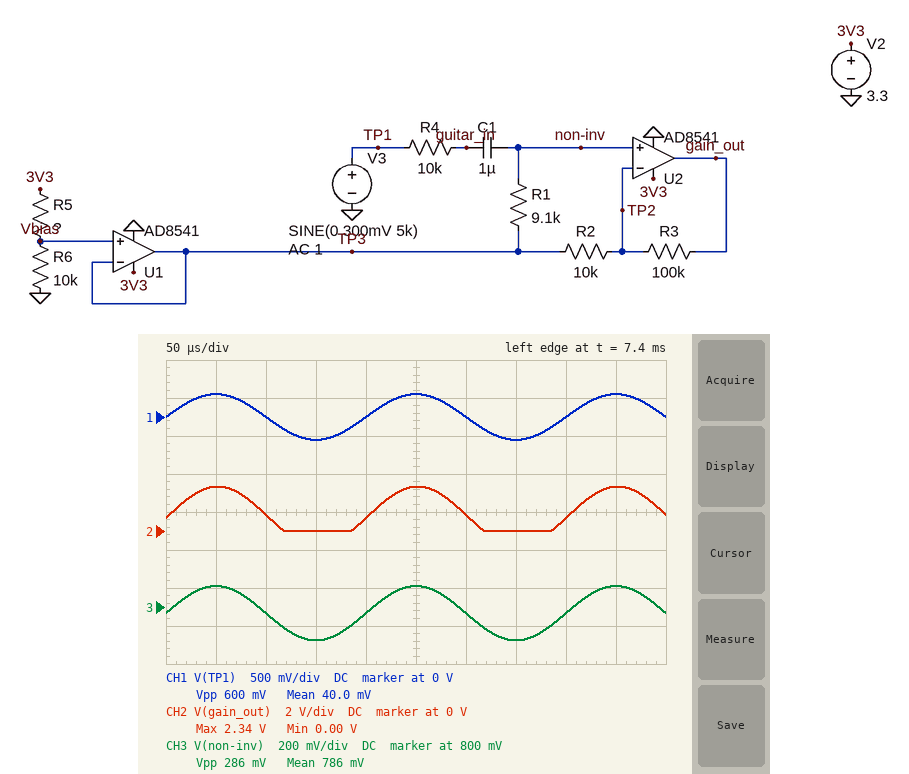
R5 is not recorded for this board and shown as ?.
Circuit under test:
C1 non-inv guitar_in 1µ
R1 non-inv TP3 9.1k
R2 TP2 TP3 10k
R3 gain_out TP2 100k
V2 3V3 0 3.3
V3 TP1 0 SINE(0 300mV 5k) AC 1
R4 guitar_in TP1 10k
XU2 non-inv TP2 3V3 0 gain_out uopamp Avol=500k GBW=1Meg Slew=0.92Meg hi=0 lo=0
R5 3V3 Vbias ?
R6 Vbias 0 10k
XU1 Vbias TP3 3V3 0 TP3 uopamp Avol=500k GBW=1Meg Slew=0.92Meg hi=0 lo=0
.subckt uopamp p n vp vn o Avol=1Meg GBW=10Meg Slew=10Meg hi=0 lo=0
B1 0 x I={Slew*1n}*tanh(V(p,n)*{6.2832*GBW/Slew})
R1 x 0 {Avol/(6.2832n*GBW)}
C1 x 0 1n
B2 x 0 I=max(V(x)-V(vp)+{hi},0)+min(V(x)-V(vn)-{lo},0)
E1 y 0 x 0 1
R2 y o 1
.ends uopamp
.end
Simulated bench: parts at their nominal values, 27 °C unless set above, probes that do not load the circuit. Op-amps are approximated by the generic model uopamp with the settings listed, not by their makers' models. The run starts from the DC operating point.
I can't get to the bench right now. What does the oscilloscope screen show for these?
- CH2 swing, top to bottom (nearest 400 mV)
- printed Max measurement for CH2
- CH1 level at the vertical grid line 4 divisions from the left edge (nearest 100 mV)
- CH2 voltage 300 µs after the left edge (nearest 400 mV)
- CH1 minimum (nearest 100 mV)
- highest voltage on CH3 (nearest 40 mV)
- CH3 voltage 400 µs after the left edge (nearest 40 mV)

2.4 V
2.34 V
0 V
800 mV
-300 mV
920 mV
760 mV
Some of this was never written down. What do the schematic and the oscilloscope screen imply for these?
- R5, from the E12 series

33 kΩ
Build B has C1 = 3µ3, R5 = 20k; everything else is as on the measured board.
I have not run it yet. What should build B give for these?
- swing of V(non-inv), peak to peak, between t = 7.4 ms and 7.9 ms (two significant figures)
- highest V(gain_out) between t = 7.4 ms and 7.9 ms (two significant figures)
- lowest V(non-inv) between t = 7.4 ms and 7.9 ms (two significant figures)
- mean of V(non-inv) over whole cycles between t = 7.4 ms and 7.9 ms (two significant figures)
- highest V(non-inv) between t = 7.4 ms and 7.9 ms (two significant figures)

290 mV
2.7 V
960 mV
1.1 V
1.2 V
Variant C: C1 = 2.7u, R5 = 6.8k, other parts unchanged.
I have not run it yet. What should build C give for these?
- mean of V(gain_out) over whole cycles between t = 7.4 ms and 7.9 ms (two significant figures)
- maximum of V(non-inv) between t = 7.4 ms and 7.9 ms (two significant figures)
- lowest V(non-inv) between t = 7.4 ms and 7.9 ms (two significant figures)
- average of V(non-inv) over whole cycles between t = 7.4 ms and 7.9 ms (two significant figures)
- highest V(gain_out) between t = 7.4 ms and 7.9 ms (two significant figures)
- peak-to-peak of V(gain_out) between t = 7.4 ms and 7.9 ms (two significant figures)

1.9 V
2.1 V
1.8 V
2.0 V
3.3 V
2.9 V
